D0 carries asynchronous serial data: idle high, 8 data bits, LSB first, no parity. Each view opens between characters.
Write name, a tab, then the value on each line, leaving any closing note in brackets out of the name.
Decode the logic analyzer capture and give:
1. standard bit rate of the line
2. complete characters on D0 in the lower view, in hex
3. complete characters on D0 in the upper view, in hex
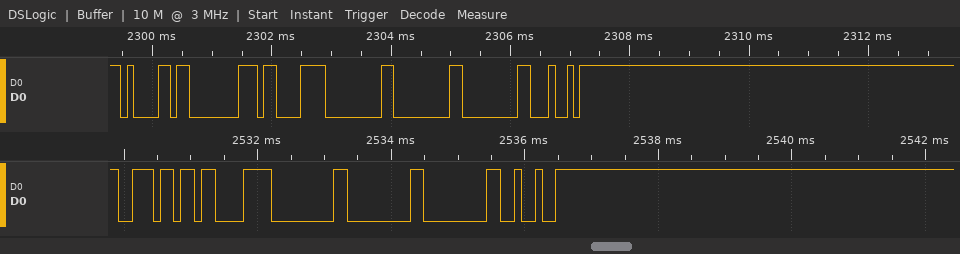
standard bit rate of the line	9600 baud
complete characters on D0 in the lower view, in hex	6E, C3, 00, 00, 00, 92
complete characters on D0 in the upper view, in hex	61, 80, C3, 00, 00, 00, A4
